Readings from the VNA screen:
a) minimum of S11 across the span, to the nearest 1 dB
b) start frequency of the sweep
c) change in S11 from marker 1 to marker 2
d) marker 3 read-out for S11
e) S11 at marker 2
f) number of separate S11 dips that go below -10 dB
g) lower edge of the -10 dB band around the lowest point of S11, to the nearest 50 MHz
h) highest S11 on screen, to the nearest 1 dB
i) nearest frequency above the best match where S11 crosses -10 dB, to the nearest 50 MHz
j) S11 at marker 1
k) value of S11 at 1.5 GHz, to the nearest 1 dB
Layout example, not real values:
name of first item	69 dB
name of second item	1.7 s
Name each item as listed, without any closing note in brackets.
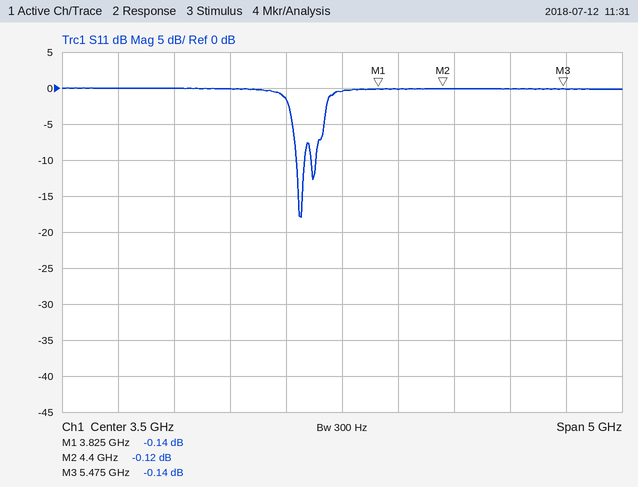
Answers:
minimum of S11 across the span, to the nearest 1 dB	-18 dB
start frequency of the sweep	1 GHz
change in S11 from marker 1 to marker 2	0.02 dB
marker 3 read-out for S11	-0.14 dB
S11 at marker 2	-0.12 dB
number of separate S11 dips that go below -10 dB	2
lower edge of the -10 dB band around the lowest point of S11, to the nearest 50 MHz	3.10 GHz
highest S11 on screen, to the nearest 1 dB	0 dB
nearest frequency above the best match where S11 crosses -10 dB, to the nearest 50 MHz	3.15 GHz
S11 at marker 1	-0.14 dB
value of S11 at 1.5 GHz, to the nearest 1 dB	0 dB
